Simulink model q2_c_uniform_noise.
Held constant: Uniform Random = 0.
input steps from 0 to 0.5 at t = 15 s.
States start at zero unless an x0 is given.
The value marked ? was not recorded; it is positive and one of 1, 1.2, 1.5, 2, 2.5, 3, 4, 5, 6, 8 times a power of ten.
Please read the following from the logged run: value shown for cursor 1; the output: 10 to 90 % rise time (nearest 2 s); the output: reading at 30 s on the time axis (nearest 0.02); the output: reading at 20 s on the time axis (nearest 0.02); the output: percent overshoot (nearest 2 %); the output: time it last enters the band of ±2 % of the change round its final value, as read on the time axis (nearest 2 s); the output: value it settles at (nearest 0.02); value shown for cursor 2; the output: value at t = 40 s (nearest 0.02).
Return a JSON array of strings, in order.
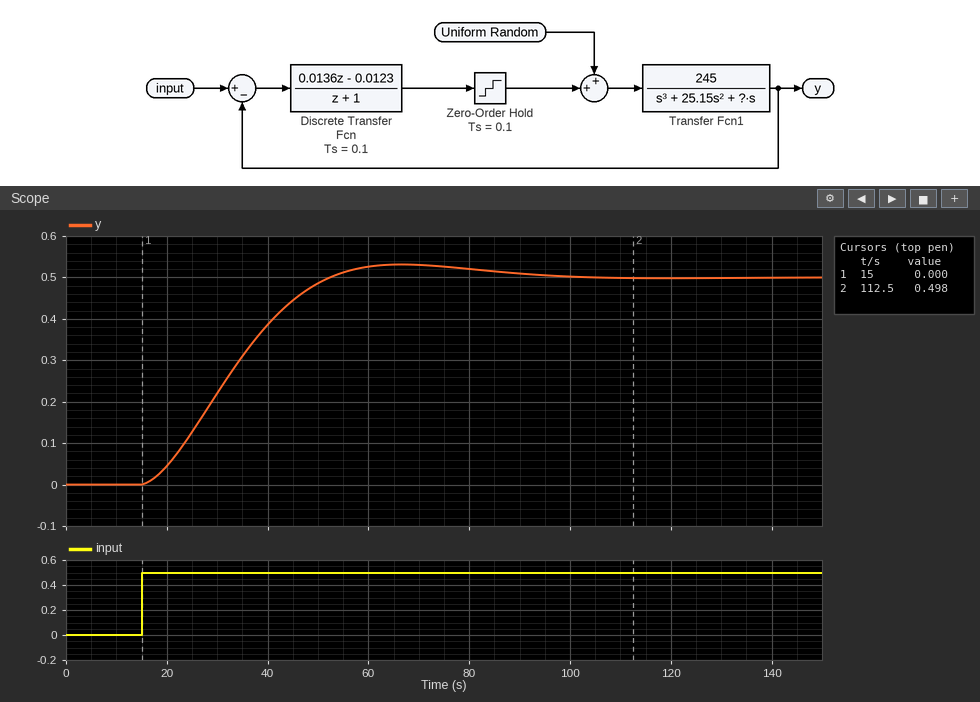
["0.000", "26 s", "0.22", "0.04", "6 %", "90 s", "0.50", "0.498", "0.38"]
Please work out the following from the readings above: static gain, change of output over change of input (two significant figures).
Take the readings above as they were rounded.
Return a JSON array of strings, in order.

["1.0"]
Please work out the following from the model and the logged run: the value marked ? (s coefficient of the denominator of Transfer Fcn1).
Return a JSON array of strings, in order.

["2.5"]
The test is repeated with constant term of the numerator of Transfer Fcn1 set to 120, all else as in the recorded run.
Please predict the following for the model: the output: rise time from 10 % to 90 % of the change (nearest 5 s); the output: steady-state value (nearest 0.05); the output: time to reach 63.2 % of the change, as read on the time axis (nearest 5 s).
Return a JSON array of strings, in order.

["55 s", "0.50", "50 s"]
